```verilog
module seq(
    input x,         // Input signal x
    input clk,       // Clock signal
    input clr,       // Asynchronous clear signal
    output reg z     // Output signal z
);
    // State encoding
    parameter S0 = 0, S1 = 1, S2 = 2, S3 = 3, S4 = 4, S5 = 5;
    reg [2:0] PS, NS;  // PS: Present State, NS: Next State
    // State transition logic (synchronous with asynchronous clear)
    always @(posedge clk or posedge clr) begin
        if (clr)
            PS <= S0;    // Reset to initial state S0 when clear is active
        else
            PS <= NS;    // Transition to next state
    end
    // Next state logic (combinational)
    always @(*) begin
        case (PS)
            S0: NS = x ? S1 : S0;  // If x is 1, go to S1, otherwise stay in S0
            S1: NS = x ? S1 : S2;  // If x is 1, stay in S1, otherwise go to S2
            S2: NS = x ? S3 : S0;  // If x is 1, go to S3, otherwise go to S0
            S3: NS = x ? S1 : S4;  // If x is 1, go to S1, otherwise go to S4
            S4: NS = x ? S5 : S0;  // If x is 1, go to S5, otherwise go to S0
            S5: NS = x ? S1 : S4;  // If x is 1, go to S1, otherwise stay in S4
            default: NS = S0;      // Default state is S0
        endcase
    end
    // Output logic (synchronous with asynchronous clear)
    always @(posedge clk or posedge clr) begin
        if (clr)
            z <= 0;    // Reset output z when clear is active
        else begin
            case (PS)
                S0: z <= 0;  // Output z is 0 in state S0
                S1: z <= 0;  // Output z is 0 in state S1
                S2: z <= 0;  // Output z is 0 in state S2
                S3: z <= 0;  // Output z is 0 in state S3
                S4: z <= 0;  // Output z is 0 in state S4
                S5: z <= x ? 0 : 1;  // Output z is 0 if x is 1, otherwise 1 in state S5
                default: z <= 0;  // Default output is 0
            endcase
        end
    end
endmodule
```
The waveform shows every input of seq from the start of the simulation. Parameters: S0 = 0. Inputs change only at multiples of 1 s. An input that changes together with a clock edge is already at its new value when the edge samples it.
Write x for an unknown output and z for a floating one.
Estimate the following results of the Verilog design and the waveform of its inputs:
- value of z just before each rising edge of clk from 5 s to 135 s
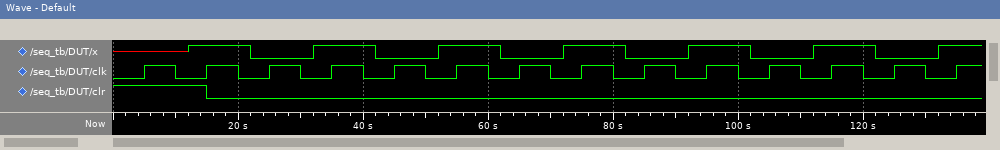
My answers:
0 0 0 0 0 0 0 1 0 1 0 1 0 1
